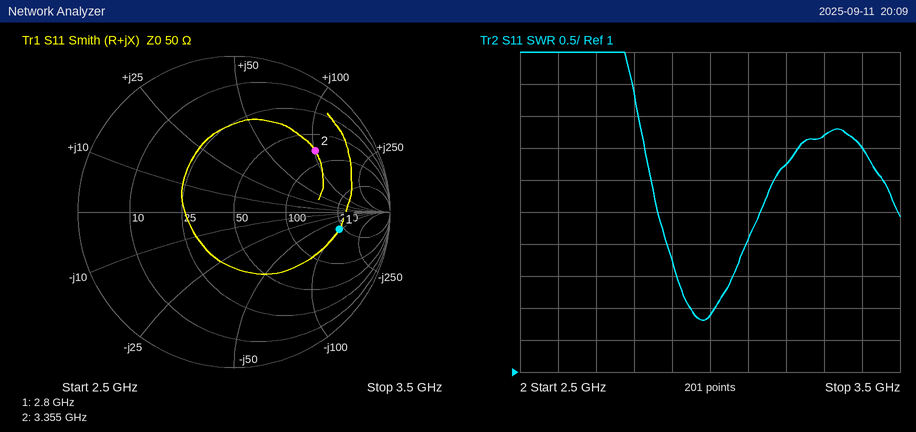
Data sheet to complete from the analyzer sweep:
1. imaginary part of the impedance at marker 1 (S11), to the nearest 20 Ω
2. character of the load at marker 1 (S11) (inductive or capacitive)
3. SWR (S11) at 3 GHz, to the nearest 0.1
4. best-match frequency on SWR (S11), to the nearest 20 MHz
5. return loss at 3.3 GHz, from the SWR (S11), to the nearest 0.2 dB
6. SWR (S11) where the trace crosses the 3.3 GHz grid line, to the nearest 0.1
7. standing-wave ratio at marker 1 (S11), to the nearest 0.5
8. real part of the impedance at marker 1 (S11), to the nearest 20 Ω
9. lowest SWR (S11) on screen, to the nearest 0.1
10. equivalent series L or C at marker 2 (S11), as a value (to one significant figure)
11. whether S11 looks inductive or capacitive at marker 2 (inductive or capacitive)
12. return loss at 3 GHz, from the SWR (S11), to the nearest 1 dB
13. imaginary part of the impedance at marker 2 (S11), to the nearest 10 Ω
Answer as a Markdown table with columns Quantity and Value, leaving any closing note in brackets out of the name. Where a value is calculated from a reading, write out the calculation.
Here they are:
| Quantity | Value |
|---|---|
| imaginary part of the impedance at marker 1 (S11), to the nearest 20 Ω | -100 Ω |
| character of the load at marker 1 (S11) | capacitive |
| SWR (S11) at 3 GHz, to the nearest 0.1 | 1.9 |
| best-match frequency on SWR (S11), to the nearest 20 MHz | 2.98 GHz |
| return loss at 3.3 GHz, from the SWR (S11), to the nearest 0.2 dB | −20 log10((4.7 − 1)/(4.7 + 1)) ≈ 3.8 dB |
| SWR (S11) where the trace crosses the 3.3 GHz grid line, to the nearest 0.1 | 4.7 |
| standing-wave ratio at marker 1 (S11), to the nearest 0.5 | 5.5 |
| real part of the impedance at marker 1 (S11), to the nearest 20 Ω | 220 Ω |
| lowest SWR (S11) on screen, to the nearest 0.1 | 1.8 |
| equivalent series L or C at marker 2 (S11), as a value | L = 100 Ω/(2π × 3.355 GHz) ≈ 5 nH |
| whether S11 looks inductive or capacitive at marker 2 | inductive |
| return loss at 3 GHz, from the SWR (S11), to the nearest 1 dB | −20 log10((1.9 − 1)/(1.9 + 1)) ≈ 10 dB |
| imaginary part of the impedance at marker 2 (S11), to the nearest 10 Ω | +100 Ω |
